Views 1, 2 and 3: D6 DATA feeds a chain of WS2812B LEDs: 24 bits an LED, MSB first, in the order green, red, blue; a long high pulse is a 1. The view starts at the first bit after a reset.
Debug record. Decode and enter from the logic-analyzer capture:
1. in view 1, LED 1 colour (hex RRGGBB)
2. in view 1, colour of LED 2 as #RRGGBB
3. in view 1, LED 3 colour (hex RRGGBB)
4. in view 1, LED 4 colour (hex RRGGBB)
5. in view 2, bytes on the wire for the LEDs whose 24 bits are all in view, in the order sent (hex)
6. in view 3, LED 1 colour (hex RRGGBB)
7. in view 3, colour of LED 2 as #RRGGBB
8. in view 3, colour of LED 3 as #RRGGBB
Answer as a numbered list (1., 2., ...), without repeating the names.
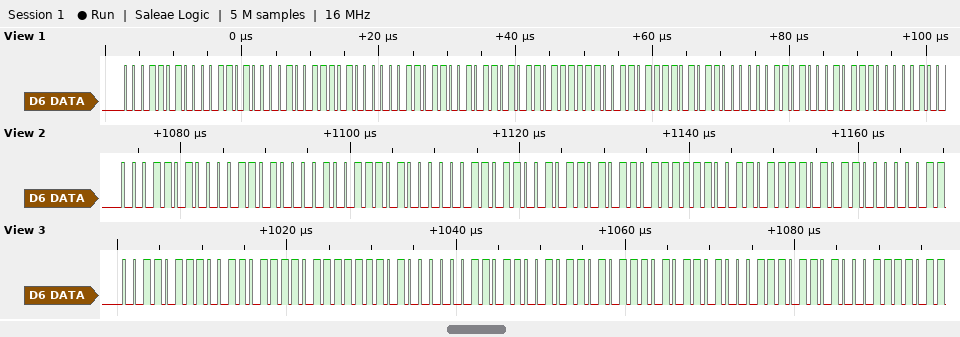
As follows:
1. #1A1A13
2. #6CA0B5
3. #37BFAC
4. #170D04
5. 1A 1A 13 A0 6C B5 BF 37 AC
6. #3737BF
7. #6CA0B5
8. #8ED6D1
